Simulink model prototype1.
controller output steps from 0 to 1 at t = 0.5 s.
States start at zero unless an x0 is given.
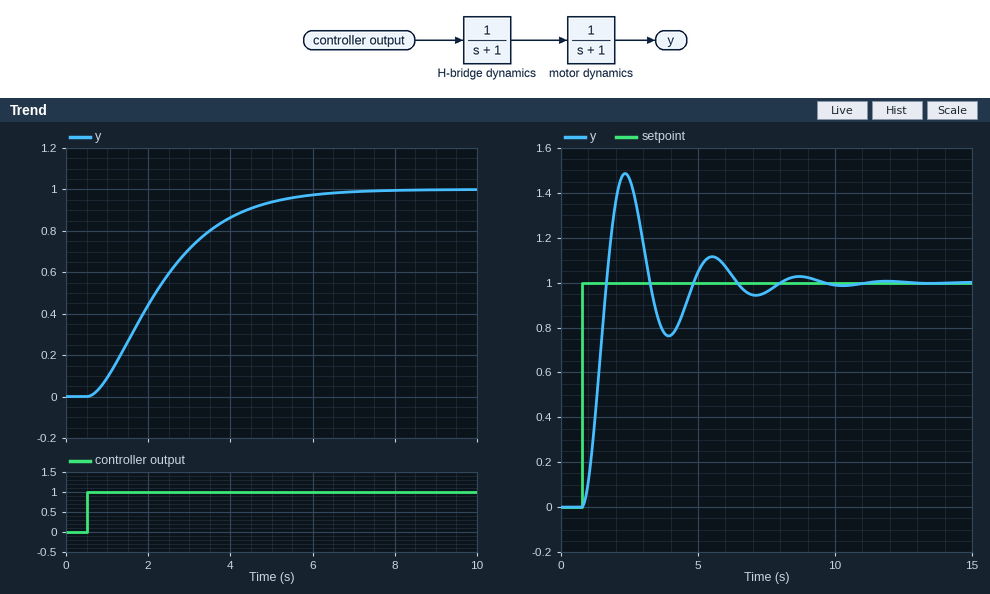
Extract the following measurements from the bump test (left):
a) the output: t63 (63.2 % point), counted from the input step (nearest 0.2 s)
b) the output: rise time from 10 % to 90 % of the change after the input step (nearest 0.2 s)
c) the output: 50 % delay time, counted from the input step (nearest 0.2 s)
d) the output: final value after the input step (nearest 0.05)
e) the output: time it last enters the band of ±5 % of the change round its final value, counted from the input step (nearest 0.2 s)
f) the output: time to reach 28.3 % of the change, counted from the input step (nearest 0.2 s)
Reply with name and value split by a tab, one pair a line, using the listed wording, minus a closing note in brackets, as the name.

the output: t63 (63.2 % point), counted from the input step	2.2 s
the output: rise time from 10 % to 90 % of the change after the input step	3.4 s
the output: 50 % delay time, counted from the input step	1.6 s
the output: final value after the input step	1.00
the output: time it last enters the band of ±5 % of the change round its final value, counted from the input step	4.8 s
the output: time to reach 28.3 % of the change, counted from the input step	1.0 s
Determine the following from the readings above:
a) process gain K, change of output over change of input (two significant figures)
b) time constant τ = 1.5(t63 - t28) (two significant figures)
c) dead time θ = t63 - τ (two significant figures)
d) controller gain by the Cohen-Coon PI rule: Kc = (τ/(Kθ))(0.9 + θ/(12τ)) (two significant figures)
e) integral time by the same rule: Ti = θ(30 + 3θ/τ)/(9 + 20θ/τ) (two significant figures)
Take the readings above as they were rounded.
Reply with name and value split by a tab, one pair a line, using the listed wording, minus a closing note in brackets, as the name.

process gain K, change of output over change of input	1.0
time constant τ = 1.5(t63 - t28)	1.8 s
dead time θ = t63 - τ	0.40 s
controller gain by the Cohen-Coon PI rule: Kc = (τ/(Kθ))(0.9 + θ/(12τ))	4.1
integral time by the same rule: Ti = θ(30 + 3θ/τ)/(9 + 20θ/τ)	0.91 s
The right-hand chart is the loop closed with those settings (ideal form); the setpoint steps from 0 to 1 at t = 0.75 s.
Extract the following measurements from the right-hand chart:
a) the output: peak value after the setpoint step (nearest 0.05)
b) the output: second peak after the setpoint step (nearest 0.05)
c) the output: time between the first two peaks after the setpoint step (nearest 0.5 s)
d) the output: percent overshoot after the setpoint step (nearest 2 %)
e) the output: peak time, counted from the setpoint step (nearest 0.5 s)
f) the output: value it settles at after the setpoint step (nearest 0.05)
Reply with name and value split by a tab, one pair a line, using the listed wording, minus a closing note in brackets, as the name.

the output: peak value after the setpoint step	1.50
the output: second peak after the setpoint step	1.10
the output: time between the first two peaks after the setpoint step	3.0 s
the output: percent overshoot after the setpoint step	48 %
the output: peak time, counted from the setpoint step	1.5 s
the output: value it settles at after the setpoint step	1.00
